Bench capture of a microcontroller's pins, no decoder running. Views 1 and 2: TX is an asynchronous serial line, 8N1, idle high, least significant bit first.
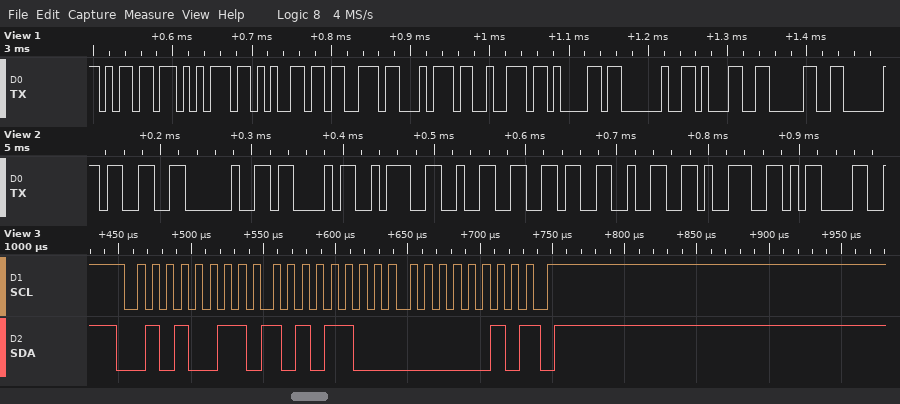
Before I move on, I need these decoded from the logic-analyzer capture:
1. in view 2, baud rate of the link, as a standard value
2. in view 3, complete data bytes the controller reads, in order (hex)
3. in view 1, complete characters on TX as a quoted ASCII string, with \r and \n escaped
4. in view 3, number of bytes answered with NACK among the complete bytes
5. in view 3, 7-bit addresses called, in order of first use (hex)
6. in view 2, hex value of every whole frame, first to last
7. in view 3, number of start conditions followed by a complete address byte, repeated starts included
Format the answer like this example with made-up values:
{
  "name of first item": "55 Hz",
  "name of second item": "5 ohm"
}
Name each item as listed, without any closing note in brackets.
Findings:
{
  "in view 2, baud rate of the link, as a standard value": "115200 baud",
  "in view 3, complete data bytes the controller reads, in order": "AC 02",
  "in view 1, complete characters on TX as a quoted ASCII string, with \\r and \\n escaped": "\"muestra 10\"",
  "in view 3, number of bytes answered with NACK among the complete bytes": "1",
  "in view 3, 7-bit addresses called, in order of first use": "0x29",
  "in view 2, hex value of every whole frame, first to last": "33 20 43 3A 32 36 32 39 0D",
  "in view 3, number of start conditions followed by a complete address byte, repeated starts included": "1"
}
